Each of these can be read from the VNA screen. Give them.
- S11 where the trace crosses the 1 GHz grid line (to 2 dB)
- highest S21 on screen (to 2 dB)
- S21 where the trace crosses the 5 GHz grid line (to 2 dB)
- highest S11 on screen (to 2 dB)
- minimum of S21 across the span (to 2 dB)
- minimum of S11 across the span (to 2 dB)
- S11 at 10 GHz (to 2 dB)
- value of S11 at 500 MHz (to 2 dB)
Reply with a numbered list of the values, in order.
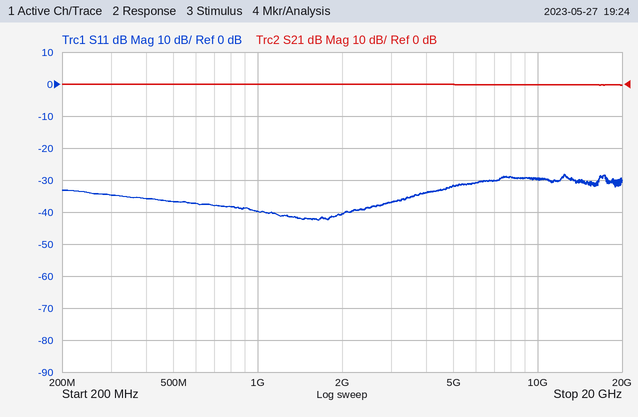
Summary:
1. -40 dB
2. 0 dB
3. 0 dB
4. -28 dB
5. 0 dB
6. -42 dB
7. -30 dB
8. -36 dB
